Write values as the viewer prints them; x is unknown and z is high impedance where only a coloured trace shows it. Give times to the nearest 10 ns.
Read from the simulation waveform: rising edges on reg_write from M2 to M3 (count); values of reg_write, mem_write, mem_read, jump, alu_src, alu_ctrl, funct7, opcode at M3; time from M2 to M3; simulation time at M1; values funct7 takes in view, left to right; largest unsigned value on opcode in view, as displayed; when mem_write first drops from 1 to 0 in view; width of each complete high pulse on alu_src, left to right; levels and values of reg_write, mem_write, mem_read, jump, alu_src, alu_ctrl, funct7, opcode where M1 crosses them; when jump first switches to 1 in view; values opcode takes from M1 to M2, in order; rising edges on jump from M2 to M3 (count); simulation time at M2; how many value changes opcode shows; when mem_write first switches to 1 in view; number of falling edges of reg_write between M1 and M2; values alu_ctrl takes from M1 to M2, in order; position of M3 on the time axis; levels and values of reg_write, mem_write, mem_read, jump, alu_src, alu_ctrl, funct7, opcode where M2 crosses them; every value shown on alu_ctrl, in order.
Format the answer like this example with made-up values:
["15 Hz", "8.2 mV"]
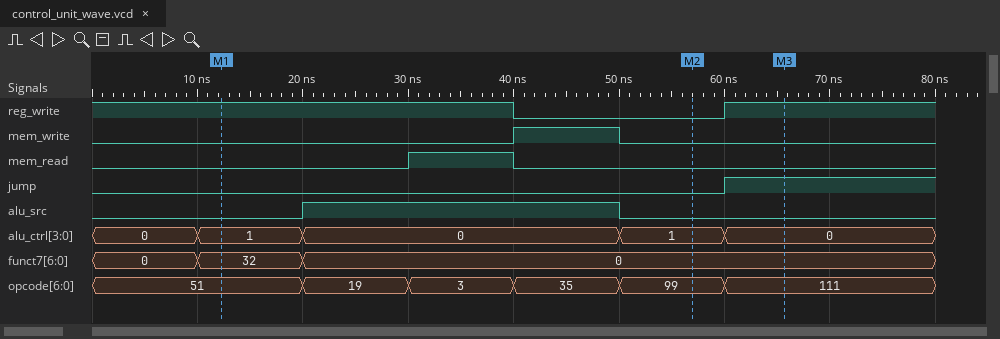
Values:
["1", "reg_write=1, mem_write=0, mem_read=0, jump=1, alu_src=0, alu_ctrl=0, funct7=0, opcode=111", "10 ns", "10 ns", "0, 32, 0", "111", "50 ns", "30 ns", "reg_write=1, mem_write=0, mem_read=0, jump=0, alu_src=0, alu_ctrl=1, funct7=32, opcode=51", "60 ns", "51, 19, 3, 35, 99", "1", "60 ns", "5", "40 ns", "1", "1, 0, 1", "70 ns", "reg_write=0, mem_write=0, mem_read=0, jump=0, alu_src=0, alu_ctrl=1, funct7=0, opcode=99", "0, 1, 0, 1, 0"]
